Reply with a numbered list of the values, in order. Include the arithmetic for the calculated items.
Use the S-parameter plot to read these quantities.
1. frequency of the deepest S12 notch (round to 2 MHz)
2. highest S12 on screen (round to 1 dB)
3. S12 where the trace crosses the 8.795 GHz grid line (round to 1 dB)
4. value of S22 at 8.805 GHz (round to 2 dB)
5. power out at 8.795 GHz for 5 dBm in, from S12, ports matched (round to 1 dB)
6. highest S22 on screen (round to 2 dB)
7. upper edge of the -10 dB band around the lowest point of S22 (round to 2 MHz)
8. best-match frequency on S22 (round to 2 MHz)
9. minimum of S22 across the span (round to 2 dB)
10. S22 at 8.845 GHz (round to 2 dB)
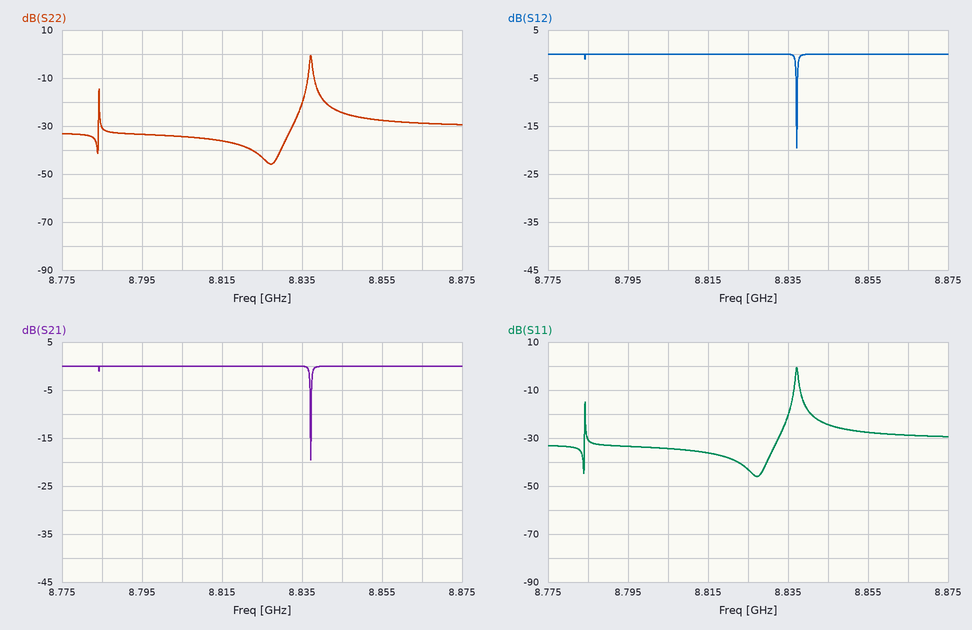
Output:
1. 8.838 GHz
2. 0 dB
3. 0 dB
4. -34 dB
5. 5 dBm + (0 dB) = 5 dBm
6. 0 dB
7. 8.836 GHz
8. 8.828 GHz
9. -46 dB
10. -24 dB
